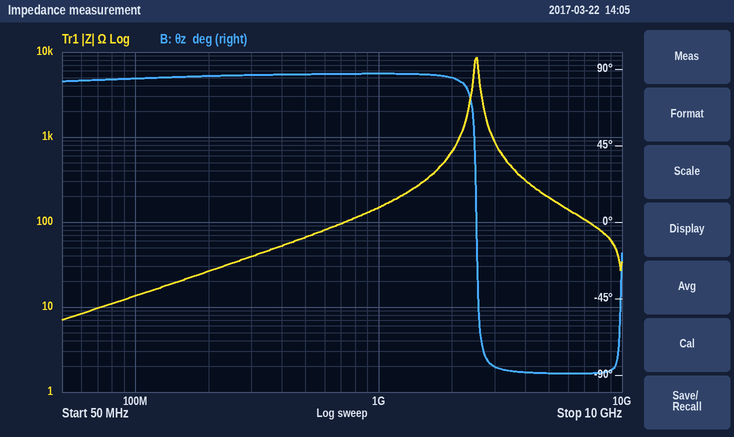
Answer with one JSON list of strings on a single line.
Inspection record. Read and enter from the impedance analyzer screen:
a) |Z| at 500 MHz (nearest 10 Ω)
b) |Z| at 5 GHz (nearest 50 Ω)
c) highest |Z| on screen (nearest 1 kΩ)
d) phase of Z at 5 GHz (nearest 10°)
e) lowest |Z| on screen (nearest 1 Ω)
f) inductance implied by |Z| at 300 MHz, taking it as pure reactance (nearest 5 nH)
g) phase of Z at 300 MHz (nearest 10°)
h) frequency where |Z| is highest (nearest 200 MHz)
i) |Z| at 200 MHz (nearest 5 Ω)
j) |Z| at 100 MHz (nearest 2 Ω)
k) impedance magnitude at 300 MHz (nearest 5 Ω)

["70 Ω", "200 Ω", "9 kΩ", "-90°", "7 Ω", "20 nH", "90°", "2.6 GHz", "25 Ω", "14 Ω", "40 Ω"]
